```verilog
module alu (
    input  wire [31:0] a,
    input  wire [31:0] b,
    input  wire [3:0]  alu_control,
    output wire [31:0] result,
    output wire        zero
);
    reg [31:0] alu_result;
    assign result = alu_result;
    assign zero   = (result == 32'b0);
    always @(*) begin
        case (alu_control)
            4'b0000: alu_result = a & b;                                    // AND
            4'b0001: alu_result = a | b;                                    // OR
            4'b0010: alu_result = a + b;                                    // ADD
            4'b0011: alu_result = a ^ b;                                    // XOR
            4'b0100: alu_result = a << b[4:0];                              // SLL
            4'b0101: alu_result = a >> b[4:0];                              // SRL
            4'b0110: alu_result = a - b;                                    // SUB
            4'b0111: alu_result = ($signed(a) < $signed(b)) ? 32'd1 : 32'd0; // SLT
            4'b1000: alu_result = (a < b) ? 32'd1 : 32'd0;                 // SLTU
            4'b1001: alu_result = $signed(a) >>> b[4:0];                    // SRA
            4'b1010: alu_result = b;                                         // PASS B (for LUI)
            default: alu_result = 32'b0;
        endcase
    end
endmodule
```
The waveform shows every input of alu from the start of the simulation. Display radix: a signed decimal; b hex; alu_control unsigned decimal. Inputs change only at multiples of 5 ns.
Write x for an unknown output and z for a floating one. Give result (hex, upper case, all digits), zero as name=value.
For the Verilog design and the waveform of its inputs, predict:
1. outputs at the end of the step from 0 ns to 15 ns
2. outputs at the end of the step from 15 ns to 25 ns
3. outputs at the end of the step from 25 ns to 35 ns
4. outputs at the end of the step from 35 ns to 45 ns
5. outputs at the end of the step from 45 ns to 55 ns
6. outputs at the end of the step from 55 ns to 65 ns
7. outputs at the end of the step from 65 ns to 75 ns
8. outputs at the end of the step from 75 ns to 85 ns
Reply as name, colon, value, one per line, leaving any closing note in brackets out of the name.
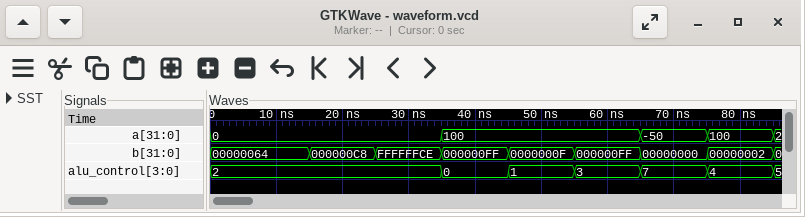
outputs at the end of the step from 0 ns to 15 ns: result=00000064, zero=0
outputs at the end of the step from 15 ns to 25 ns: result=000000C8, zero=0
outputs at the end of the step from 25 ns to 35 ns: result=FFFFFFCE, zero=0
outputs at the end of the step from 35 ns to 45 ns: result=00000064, zero=0
outputs at the end of the step from 45 ns to 55 ns: result=0000006F, zero=0
outputs at the end of the step from 55 ns to 65 ns: result=0000009B, zero=0
outputs at the end of the step from 65 ns to 75 ns: result=00000001, zero=0
outputs at the end of the step from 75 ns to 85 ns: result=00000190, zero=0
